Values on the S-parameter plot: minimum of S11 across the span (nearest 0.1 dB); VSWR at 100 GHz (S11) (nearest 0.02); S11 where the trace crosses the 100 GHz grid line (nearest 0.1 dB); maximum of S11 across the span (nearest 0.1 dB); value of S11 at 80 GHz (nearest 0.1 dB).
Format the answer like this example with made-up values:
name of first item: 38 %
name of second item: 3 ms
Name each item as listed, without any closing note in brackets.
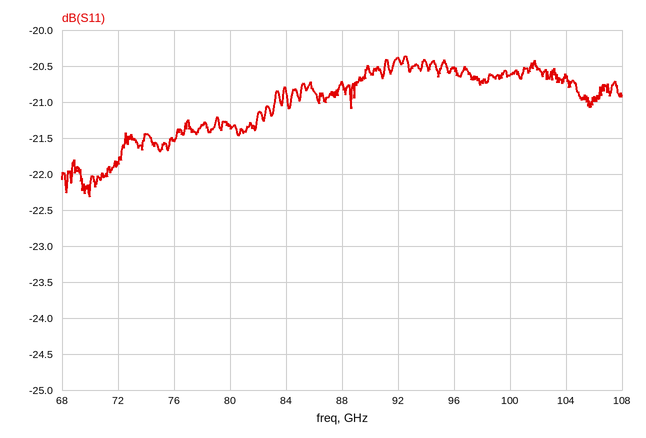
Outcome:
minimum of S11 across the span: -22.3 dB
VSWR at 100 GHz (S11): 1.20
S11 where the trace crosses the 100 GHz grid line: -20.6 dB
maximum of S11 across the span: -20.4 dB
value of S11 at 80 GHz: -21.3 dB
